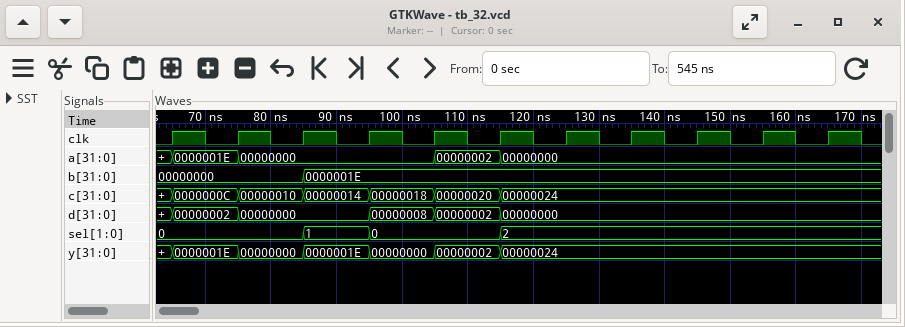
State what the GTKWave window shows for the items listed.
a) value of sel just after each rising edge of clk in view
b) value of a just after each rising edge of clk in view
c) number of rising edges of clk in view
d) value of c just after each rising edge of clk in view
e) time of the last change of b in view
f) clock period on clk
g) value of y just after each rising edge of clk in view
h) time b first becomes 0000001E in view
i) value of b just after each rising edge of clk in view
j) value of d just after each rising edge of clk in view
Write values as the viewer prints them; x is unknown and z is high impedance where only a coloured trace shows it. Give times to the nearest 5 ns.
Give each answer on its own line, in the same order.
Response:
0, 0, 1, 0, 0, 2, 2, 2, 2, 2, 2
0000001E, 00000000, 00000000, 00000000, 00000002, 00000000, 00000000, 00000000, 00000000, 00000000, 00000000
11
0000000C, 00000010, 00000014, 00000018, 00000020, 00000024, 00000024, 00000024, 00000024, 00000024, 00000024
85 ns
10 ns
0000001E, 00000000, 0000001E, 00000000, 00000002, 00000024, 00000024, 00000024, 00000024, 00000024, 00000024
85 ns
00000000, 00000000, 0000001E, 0000001E, 0000001E, 0000001E, 0000001E, 0000001E, 0000001E, 0000001E, 0000001E
00000002, 00000000, 00000000, 00000008, 00000002, 00000000, 00000000, 00000000, 00000000, 00000000, 00000000
